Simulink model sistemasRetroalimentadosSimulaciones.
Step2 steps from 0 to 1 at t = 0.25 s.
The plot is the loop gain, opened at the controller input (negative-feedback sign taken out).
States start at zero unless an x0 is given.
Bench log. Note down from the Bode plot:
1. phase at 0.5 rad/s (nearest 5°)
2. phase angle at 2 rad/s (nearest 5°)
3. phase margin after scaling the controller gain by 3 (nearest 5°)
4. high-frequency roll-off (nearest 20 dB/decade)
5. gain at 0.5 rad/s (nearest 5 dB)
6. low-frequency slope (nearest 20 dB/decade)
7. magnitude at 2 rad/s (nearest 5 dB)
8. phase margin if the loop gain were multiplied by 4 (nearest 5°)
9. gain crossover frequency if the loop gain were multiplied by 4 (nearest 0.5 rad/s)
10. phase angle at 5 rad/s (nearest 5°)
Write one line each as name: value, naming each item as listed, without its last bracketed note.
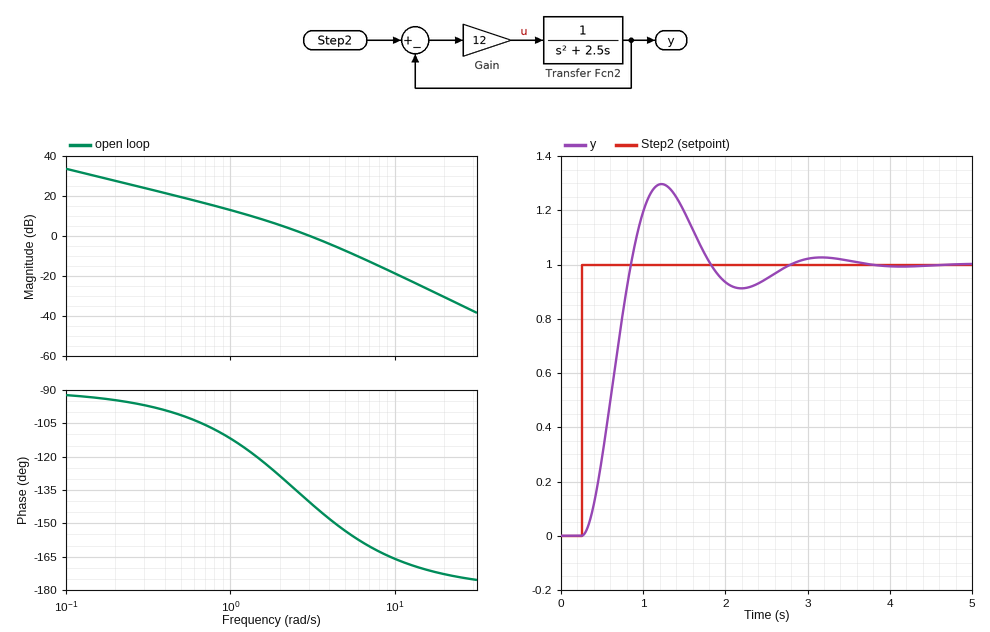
phase at 0.5 rad/s: -100°
phase angle at 2 rad/s: -130°
phase margin after scaling the controller gain by 3: 25°
high-frequency roll-off: -40 dB/decade
gain at 0.5 rad/s: 20 dB
low-frequency slope: -20 dB/decade
magnitude at 2 rad/s: 5 dB
phase margin if the loop gain were multiplied by 4: 20°
gain crossover frequency if the loop gain were multiplied by 4: 6.5 rad/s
phase angle at 5 rad/s: -155°
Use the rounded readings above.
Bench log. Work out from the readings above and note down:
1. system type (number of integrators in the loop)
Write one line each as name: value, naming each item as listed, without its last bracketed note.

system type: 1
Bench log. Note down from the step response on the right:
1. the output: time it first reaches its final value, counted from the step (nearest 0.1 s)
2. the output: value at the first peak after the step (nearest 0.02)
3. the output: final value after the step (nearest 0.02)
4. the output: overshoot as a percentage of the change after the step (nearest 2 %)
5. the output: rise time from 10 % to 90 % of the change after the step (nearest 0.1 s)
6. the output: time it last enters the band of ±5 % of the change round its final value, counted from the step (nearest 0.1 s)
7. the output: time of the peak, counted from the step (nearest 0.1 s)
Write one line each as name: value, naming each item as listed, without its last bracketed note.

the output: time it first reaches its final value, counted from the step: 0.6 s
the output: value at the first peak after the step: 1.30
the output: final value after the step: 1.00
the output: overshoot as a percentage of the change after the step: 30 %
the output: rise time from 10 % to 90 % of the change after the step: 0.4 s
the output: time it last enters the band of ±5 % of the change round its final value, counted from the step: 2.3 s
the output: time of the peak, counted from the step: 1.0 s
